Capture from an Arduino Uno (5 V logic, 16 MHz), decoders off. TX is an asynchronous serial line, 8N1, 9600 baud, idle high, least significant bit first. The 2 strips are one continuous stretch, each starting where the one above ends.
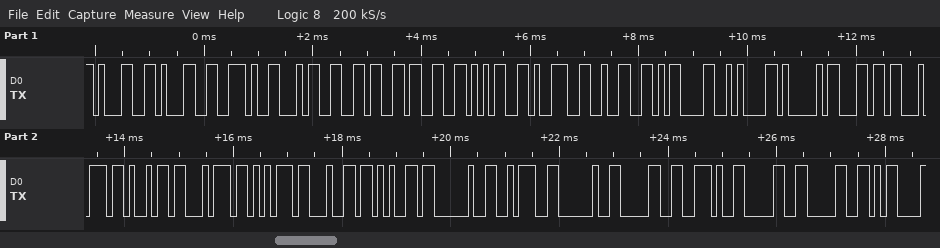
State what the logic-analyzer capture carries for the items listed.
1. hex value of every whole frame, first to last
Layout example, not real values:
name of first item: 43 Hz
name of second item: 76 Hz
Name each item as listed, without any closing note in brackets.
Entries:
hex value of every whole frame, first to last: 31 31 2E 34 36 33 35 39 32 0D 0A 41 6C 74 69 74 75 64 65 20 3A 20 30 2E 30 30 0D
